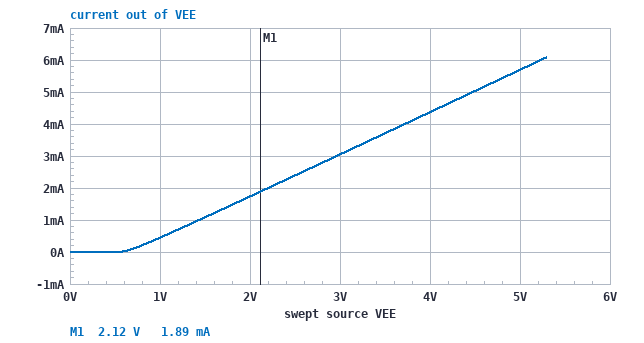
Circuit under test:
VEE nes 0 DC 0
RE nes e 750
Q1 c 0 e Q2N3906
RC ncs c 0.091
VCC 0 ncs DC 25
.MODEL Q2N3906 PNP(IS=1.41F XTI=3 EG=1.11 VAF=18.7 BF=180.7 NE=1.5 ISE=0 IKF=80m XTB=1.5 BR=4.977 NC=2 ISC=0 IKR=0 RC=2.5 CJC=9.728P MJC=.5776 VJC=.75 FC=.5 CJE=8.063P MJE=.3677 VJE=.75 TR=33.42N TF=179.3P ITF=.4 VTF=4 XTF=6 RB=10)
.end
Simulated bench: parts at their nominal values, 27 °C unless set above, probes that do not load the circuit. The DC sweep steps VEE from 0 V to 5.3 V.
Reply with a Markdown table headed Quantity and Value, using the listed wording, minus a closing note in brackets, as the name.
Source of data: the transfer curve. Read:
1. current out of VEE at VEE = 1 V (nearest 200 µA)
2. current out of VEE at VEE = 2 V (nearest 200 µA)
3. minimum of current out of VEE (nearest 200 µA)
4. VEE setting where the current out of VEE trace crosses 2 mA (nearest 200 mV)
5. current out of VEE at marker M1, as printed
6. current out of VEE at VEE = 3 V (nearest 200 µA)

| Quantity | Value |
|---|---|
| current out of VEE at VEE = 1 V | 400 µA |
| current out of VEE at VEE = 2 V | 1.8 mA |
| minimum of current out of VEE | 0 A |
| VEE setting where the current out of VEE trace crosses 2 mA | 2.2 V |
| current out of VEE at marker M1, as printed | 1.89 mA |
| current out of VEE at VEE = 3 V | 3.0 mA |
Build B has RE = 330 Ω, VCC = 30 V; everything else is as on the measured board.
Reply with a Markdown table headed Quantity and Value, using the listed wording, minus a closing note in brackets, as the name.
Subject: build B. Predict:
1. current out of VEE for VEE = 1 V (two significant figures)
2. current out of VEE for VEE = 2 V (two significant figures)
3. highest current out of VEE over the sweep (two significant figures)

| Quantity | Value |
|---|---|
| current out of VEE for VEE = 1 V | 970 µA |
| current out of VEE for VEE = 2 V | 3.9 mA |
| highest current out of VEE over the sweep | 14 mA |
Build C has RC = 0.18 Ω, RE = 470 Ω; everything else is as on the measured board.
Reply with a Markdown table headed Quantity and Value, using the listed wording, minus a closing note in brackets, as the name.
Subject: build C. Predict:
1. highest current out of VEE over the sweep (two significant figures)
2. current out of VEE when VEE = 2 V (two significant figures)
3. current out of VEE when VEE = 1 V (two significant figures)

| Quantity | Value |
|---|---|
| highest current out of VEE over the sweep | 9.7 mA |
| current out of VEE when VEE = 2 V | 2.7 mA |
| current out of VEE when VEE = 1 V | 690 µA |
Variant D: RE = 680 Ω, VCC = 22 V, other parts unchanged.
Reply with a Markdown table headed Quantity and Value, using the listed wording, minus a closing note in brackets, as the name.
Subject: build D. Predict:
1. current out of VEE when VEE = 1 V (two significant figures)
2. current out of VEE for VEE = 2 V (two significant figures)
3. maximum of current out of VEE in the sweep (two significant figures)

| Quantity | Value |
|---|---|
| current out of VEE when VEE = 1 V | 490 µA |
| current out of VEE for VEE = 2 V | 1.9 mA |
| maximum of current out of VEE in the sweep | 6.7 mA |
